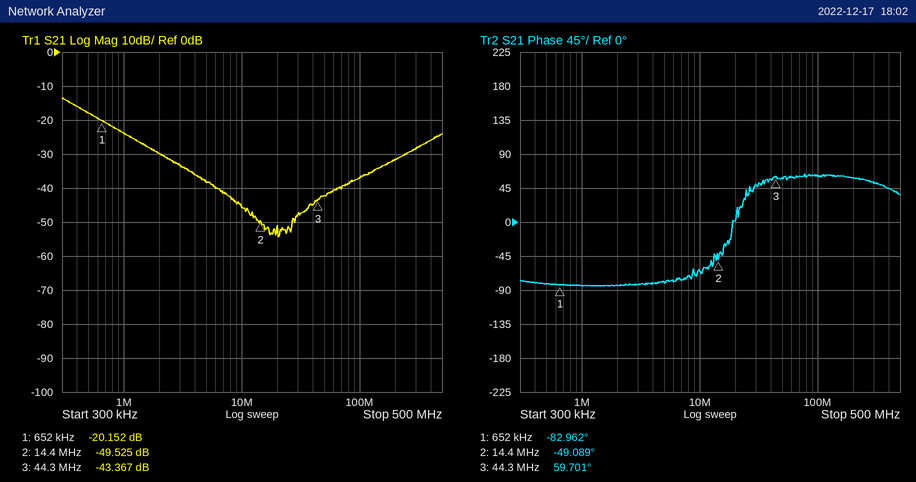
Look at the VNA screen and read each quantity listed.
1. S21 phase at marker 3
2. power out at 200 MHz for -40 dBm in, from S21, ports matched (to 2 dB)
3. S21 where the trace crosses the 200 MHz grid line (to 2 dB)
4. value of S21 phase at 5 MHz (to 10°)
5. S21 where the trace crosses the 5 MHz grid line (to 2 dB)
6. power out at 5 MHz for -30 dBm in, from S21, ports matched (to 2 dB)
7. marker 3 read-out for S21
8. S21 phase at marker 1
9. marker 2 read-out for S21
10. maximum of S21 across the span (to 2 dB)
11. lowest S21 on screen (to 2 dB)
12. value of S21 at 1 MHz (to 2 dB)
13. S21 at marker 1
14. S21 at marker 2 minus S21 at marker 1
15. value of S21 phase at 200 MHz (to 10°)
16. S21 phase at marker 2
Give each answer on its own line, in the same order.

59.701°
-72 dBm
-32 dB
-80°
-38 dB
-68 dBm
-43.367 dB
-82.962°
-49.525 dB
-14 dB
-54 dB
-24 dB
-20.152 dB
-29.373 dB
60°
-49.089°
